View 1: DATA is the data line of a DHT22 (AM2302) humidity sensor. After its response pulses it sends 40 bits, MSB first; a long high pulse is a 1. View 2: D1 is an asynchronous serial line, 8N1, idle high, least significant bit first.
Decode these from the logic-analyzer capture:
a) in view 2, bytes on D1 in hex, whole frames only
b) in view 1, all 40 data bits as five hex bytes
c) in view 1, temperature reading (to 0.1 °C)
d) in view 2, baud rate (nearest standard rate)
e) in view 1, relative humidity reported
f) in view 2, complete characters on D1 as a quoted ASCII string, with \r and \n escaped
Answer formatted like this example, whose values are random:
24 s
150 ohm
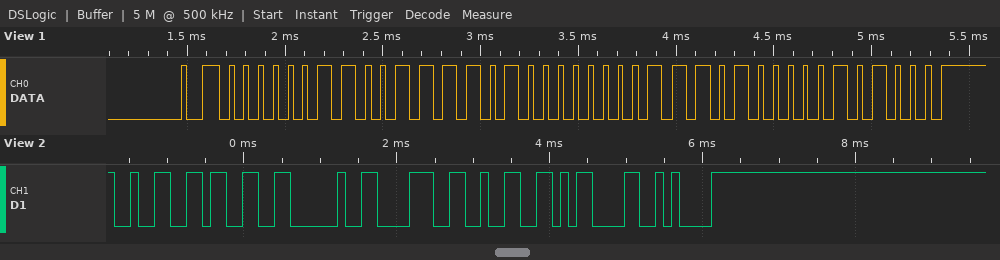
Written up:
32 33 20 38 32 0D 0A
03 3D 00 E8 28
23.2 °C
9600 baud
82.9 %
"23 82\r\n"
